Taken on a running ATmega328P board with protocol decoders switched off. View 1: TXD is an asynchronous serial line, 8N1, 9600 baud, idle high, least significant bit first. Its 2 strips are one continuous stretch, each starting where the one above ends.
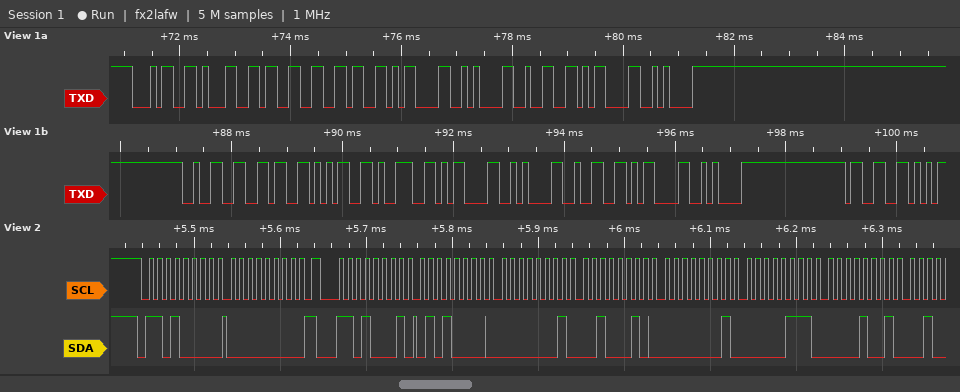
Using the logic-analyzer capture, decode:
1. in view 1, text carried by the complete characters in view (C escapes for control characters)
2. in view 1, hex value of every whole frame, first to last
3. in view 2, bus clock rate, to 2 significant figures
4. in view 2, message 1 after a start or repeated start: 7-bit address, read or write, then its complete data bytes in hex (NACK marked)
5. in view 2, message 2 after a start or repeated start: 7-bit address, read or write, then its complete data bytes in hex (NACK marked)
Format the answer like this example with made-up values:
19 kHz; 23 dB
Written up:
"4136\r\n2\r\n2659\r\n2\r\n3"; 34 31 33 36 0D 0A 32 0D 0A 32 36 35 39 0D 0A 32 0D 0A 33; 100 kHz; 0x68 write: 00; 0x68 read: 50 01 22 01 07 09
